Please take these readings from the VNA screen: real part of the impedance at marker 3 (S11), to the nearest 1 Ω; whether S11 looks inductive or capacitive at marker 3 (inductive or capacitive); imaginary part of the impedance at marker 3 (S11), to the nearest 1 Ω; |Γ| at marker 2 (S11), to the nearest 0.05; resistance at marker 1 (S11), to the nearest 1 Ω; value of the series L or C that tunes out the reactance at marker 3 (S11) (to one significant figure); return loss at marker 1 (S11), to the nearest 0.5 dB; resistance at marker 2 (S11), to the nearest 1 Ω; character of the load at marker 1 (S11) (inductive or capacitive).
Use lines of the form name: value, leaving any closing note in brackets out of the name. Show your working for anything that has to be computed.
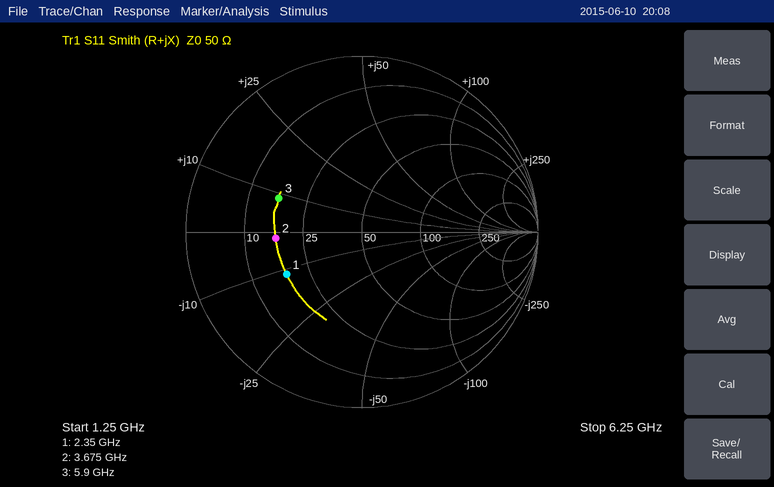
real part of the impedance at marker 3 (S11), to the nearest 1 Ω: 17 Ω
whether S11 looks inductive or capacitive at marker 3: inductive
imaginary part of the impedance at marker 3 (S11), to the nearest 1 Ω: +9 Ω
|Γ| at marker 2 (S11), to the nearest 0.05: 0.50
resistance at marker 1 (S11), to the nearest 1 Ω: 18 Ω
value of the series L or C that tunes out the reactance at marker 3 (S11): C = 1/(2π × 5.9 GHz × 9 Ω) ≈ 3 pF
return loss at marker 1 (S11), to the nearest 0.5 dB: 6.0 dB
resistance at marker 2 (S11), to the nearest 1 Ω: 17 Ω
character of the load at marker 1 (S11): capacitive
